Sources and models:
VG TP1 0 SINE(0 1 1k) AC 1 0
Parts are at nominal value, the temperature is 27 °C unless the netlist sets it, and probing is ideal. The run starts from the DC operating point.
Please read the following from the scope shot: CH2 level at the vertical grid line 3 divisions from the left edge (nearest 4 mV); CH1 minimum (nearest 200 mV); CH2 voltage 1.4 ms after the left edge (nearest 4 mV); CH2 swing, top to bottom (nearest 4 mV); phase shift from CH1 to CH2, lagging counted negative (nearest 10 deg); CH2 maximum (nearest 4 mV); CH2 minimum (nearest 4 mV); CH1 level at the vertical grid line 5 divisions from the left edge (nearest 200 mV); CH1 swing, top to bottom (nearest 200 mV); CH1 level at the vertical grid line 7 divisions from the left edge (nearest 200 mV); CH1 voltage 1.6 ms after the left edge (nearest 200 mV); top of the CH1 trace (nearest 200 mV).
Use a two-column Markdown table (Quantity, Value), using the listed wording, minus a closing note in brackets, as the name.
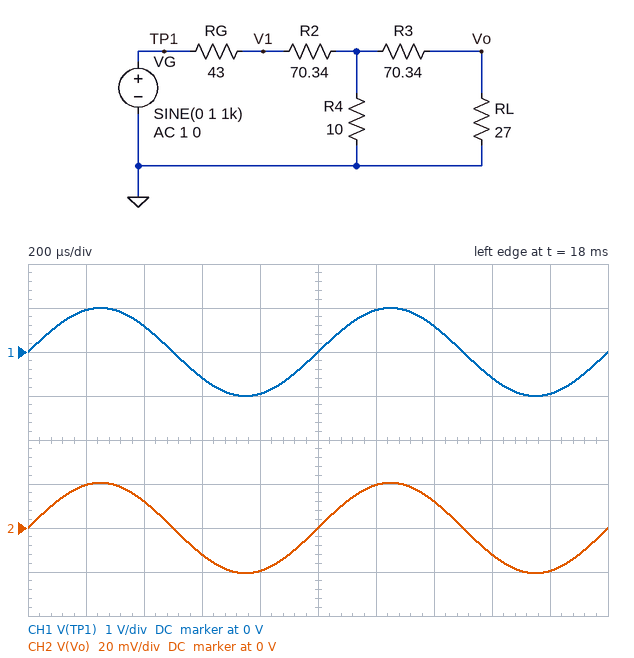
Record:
| Quantity | Value |
|---|---|
| CH2 level at the vertical grid line 3 divisions from the left edge | -12 mV |
| CH1 minimum | -1.0 V |
| CH2 voltage 1.4 ms after the left edge | 12 mV |
| CH2 swing, top to bottom | 40 mV |
| phase shift from CH1 to CH2, lagging counted negative | 0 deg |
| CH2 maximum | 20 mV |
| CH2 minimum | -20 mV |
| CH1 level at the vertical grid line 5 divisions from the left edge | 0 V |
| CH1 swing, top to bottom | 2.0 V |
| CH1 level at the vertical grid line 7 divisions from the left edge | 600 mV |
| CH1 voltage 1.6 ms after the left edge | -600 mV |
| top of the CH1 trace | 1.0 V |
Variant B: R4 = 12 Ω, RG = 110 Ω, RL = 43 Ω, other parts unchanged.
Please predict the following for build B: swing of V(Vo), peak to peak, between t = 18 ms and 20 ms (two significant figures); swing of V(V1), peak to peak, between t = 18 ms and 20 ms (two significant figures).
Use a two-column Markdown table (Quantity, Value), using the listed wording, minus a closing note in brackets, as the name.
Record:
| Quantity | Value |
|---|---|
| swing of V(Vo), peak to peak, between t = 18 ms and 20 ms | 43 mV |
| swing of V(V1), peak to peak, between t = 18 ms and 20 ms | 850 mV |
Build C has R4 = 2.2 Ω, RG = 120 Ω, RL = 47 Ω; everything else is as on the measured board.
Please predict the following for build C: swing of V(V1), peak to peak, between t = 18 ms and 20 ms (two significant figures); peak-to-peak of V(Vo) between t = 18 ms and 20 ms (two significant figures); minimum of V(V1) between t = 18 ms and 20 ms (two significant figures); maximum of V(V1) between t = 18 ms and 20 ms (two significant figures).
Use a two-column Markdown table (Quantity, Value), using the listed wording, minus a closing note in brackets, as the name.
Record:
| Quantity | Value |
|---|---|
| swing of V(V1), peak to peak, between t = 18 ms and 20 ms | 750 mV |
| peak-to-peak of V(Vo) between t = 18 ms and 20 ms | 9.0 mV |
| minimum of V(V1) between t = 18 ms and 20 ms | -380 mV |
| maximum of V(V1) between t = 18 ms and 20 ms | 380 mV |
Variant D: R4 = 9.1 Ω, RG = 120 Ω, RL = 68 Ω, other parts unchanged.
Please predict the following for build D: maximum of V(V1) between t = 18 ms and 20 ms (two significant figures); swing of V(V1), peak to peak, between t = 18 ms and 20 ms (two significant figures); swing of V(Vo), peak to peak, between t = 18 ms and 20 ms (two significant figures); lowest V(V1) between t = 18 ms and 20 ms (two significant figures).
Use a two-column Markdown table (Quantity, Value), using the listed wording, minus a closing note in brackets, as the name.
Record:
| Quantity | Value |
|---|---|
| maximum of V(V1) between t = 18 ms and 20 ms | 400 mV |
| swing of V(V1), peak to peak, between t = 18 ms and 20 ms | 790 mV |
| swing of V(Vo), peak to peak, between t = 18 ms and 20 ms | 42 mV |
| lowest V(V1) between t = 18 ms and 20 ms | -400 mV |
